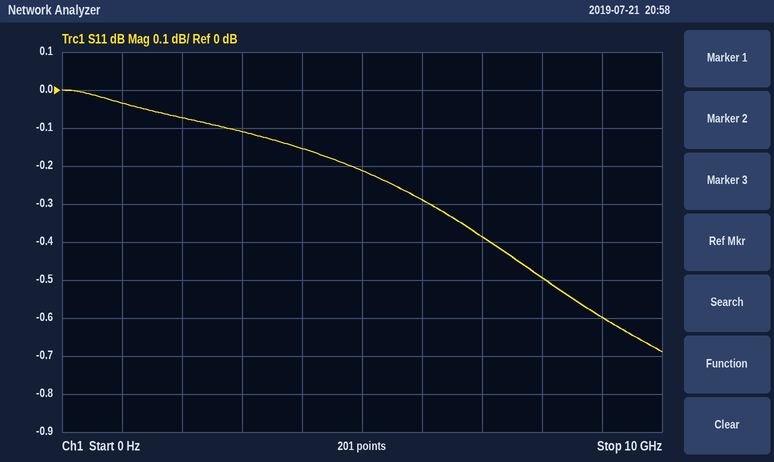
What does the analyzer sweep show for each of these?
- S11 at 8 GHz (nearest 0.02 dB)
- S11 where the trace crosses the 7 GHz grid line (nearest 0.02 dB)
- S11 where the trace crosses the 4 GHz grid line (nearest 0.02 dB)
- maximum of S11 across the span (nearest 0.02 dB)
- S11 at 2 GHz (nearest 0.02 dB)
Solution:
-0.50 dB
-0.38 dB
-0.16 dB
0.00 dB
-0.08 dB
